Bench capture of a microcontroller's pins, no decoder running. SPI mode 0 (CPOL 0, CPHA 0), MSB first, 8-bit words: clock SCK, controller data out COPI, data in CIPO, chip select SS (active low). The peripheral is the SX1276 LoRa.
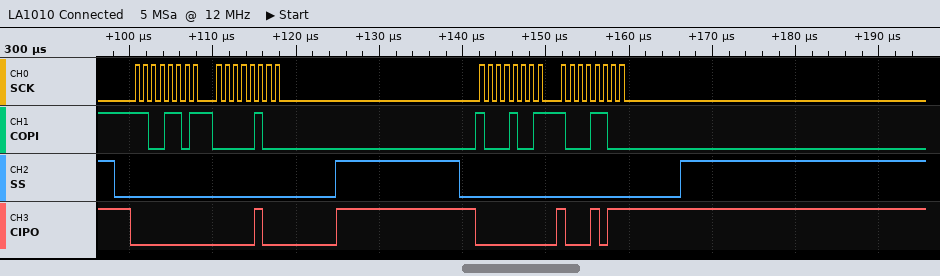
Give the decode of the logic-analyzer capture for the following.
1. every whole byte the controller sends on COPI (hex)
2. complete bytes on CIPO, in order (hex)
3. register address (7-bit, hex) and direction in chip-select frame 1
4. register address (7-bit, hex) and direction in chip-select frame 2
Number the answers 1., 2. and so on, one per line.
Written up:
1. 0xCD 0x04 0x89 0x8C
2. 0x00 0x04 0x00 0x8B
3. 0x4D write
4. 0x09 write
